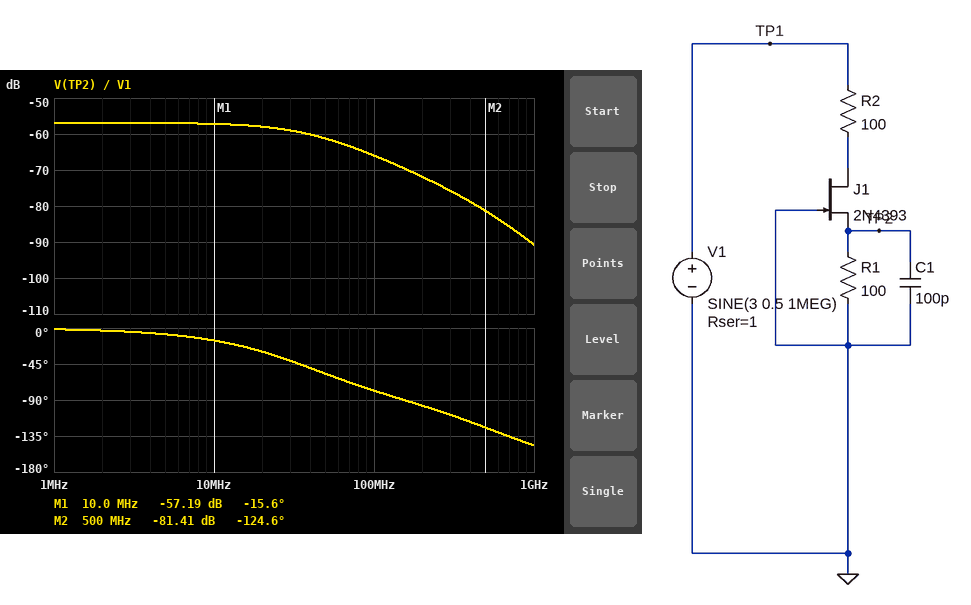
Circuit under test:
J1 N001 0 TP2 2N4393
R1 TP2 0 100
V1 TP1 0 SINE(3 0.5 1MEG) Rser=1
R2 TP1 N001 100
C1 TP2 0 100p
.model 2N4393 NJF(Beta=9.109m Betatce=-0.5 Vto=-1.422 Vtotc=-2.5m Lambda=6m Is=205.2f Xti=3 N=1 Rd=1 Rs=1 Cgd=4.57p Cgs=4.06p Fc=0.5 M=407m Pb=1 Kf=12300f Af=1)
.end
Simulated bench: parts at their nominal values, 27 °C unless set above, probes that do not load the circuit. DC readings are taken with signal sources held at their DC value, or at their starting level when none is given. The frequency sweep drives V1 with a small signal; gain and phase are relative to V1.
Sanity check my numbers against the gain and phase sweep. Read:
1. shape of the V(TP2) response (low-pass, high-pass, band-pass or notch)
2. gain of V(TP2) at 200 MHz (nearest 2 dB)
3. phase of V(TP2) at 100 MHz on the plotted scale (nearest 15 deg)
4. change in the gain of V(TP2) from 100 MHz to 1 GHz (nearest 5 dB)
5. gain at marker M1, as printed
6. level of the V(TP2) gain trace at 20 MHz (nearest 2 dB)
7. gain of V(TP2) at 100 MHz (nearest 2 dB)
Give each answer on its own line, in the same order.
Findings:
low-pass
-72 dB
-75 deg
-25 dB
-57.19 dB
-58 dB
-66 dB
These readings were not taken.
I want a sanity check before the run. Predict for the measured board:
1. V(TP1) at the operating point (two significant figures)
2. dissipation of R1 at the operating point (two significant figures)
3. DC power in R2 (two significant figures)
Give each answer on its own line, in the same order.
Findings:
3.0 V
3.7 mW
3.7 mW
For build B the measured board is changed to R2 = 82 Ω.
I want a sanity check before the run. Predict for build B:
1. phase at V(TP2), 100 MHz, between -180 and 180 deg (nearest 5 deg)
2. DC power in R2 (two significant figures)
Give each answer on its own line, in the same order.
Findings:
-75 deg
3.0 mW
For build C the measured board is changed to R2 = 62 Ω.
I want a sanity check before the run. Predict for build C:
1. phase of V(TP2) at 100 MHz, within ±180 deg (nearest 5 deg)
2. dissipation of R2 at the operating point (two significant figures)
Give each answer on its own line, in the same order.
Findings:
-75 deg
2.3 mW
